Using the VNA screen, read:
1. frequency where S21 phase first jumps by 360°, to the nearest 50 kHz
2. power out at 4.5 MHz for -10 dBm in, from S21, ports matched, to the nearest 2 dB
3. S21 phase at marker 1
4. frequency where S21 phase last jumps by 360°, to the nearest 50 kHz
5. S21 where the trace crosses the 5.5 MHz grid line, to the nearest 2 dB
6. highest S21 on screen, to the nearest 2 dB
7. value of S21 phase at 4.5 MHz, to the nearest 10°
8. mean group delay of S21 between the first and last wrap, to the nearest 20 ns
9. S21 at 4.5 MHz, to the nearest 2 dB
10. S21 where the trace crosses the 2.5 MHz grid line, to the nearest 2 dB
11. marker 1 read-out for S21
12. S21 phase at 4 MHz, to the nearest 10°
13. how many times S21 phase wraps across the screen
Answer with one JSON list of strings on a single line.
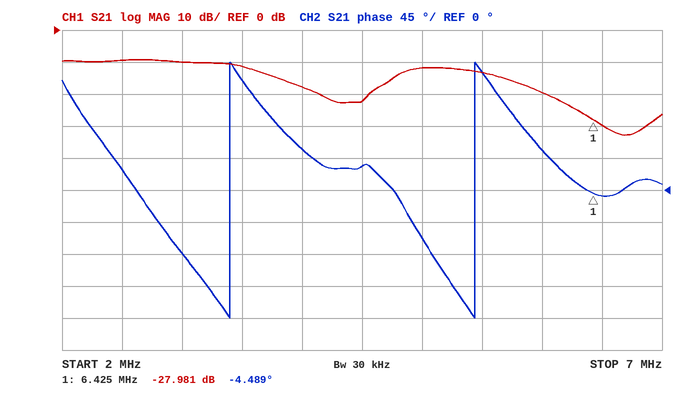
["3.40 MHz", "-32 dBm", "-4.489°", "5.45 MHz", "-14 dB", "-10 dB", "30°", "480 ns", "-22 dB", "-10 dB", "-27.981 dB", "60°", "2"]
